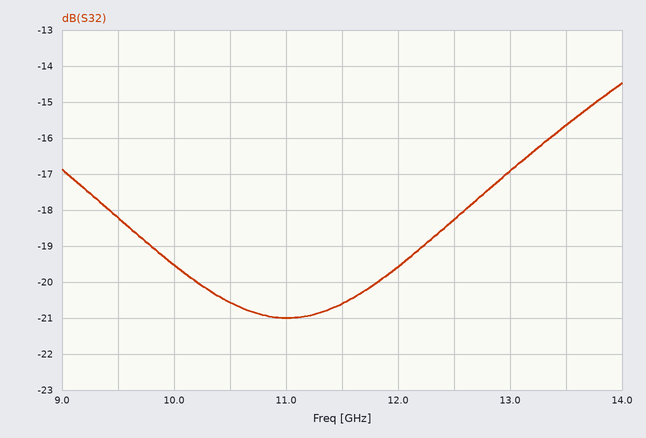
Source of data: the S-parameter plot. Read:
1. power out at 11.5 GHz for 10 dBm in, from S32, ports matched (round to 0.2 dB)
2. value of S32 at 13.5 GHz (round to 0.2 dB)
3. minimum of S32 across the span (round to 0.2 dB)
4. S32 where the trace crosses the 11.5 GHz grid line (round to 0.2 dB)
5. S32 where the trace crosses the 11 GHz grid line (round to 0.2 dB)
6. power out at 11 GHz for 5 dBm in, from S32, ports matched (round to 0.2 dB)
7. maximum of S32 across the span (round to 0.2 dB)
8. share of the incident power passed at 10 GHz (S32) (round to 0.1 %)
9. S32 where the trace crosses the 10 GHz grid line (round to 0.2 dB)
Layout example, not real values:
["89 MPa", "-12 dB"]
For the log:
["-10.6 dBm", "-15.6 dB", "-21.0 dB", "-20.6 dB", "-21.0 dB", "-16.0 dBm", "-14.4 dB", "1.1 %", "-19.6 dB"]
